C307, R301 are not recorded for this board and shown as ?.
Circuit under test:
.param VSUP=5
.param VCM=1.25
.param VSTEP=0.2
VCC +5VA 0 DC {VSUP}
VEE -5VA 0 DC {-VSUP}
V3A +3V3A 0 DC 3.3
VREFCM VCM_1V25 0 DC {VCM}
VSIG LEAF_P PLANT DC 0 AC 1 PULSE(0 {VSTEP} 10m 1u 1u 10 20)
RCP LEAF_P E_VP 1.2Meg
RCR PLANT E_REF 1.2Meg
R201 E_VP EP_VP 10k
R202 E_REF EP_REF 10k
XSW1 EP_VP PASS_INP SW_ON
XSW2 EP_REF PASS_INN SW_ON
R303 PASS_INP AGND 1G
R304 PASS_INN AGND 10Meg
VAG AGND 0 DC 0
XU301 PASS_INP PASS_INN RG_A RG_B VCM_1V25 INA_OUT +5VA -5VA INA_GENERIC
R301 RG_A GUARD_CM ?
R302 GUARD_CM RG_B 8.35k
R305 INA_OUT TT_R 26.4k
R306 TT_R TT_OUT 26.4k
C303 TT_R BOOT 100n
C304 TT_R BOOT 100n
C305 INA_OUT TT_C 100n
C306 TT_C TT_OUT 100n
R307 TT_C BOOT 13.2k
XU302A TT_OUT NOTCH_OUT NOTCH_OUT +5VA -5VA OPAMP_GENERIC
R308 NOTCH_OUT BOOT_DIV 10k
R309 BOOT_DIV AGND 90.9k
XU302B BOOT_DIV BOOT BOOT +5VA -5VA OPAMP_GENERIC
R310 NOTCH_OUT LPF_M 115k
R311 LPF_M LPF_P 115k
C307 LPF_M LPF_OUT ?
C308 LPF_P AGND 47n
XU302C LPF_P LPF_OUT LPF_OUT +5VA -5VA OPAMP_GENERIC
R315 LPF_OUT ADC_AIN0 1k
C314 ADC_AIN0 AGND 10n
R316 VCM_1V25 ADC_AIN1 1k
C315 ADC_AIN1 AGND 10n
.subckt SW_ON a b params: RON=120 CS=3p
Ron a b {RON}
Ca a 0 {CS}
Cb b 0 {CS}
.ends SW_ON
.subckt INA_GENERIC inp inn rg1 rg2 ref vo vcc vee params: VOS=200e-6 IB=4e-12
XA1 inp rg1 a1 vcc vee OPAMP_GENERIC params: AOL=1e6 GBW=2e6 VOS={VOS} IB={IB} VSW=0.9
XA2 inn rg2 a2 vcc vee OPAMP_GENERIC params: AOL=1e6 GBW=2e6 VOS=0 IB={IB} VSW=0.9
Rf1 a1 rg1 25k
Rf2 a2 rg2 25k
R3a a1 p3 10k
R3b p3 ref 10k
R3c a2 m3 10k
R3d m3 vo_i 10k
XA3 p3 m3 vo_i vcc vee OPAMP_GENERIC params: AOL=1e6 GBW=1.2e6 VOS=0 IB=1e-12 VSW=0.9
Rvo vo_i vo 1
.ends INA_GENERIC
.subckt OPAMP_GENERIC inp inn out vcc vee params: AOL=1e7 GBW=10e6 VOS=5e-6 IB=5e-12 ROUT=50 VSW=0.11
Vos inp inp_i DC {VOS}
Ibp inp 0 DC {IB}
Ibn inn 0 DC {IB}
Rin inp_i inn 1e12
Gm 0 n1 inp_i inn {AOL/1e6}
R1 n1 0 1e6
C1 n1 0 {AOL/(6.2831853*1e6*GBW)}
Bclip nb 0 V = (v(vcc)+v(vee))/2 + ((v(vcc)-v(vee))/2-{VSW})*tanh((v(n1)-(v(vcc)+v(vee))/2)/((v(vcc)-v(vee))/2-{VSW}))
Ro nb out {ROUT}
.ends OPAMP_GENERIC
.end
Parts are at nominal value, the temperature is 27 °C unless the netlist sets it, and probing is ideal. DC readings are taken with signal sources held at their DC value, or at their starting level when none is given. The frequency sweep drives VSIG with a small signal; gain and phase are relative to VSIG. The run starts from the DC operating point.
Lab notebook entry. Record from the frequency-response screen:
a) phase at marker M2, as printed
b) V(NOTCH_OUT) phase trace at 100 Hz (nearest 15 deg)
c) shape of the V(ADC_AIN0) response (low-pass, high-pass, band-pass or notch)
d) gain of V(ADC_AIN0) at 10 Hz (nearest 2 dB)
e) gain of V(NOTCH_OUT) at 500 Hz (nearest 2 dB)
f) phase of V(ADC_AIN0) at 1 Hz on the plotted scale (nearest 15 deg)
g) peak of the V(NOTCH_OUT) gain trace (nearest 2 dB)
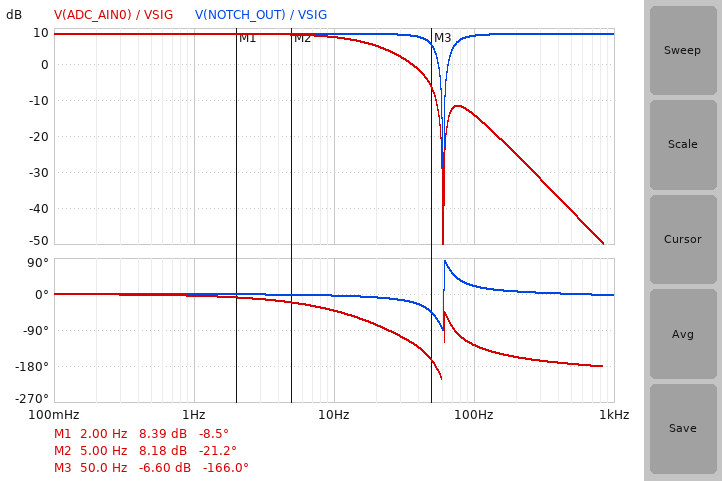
-21.2 deg
15 deg
low-pass
8 dB
8 dB
0 deg
8 dB
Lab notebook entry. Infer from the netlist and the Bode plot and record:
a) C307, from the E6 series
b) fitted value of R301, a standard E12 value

47 nF
22 kΩ
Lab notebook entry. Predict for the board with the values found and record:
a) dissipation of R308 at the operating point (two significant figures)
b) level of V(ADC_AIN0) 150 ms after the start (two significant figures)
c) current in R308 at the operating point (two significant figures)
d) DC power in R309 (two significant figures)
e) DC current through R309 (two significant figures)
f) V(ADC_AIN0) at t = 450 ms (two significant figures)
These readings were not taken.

1.5 µW
1.8 V
12 µA
14 µW
12 µA
1.8 V
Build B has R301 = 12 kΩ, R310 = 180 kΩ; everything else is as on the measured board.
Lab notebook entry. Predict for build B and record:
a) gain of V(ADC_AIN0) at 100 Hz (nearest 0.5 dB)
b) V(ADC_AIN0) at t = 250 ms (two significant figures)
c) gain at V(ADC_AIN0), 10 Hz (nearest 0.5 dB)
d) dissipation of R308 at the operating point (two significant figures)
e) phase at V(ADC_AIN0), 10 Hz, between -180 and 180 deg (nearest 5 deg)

-15.5 dB
1.9 V
9.0 dB
1.5 µW
-50 deg
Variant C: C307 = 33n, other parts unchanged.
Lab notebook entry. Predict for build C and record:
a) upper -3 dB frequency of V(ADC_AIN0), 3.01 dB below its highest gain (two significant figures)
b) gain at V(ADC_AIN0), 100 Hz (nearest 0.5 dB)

17 Hz
-12.0 dB
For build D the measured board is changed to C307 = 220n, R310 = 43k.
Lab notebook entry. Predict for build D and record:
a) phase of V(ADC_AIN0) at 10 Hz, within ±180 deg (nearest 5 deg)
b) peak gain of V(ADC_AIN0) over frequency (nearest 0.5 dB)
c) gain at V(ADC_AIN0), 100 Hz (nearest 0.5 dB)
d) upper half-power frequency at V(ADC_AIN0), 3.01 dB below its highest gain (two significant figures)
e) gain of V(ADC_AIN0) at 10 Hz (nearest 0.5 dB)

-35 deg
9.5 dB
-18.0 dB
26 Hz
9.0 dB
